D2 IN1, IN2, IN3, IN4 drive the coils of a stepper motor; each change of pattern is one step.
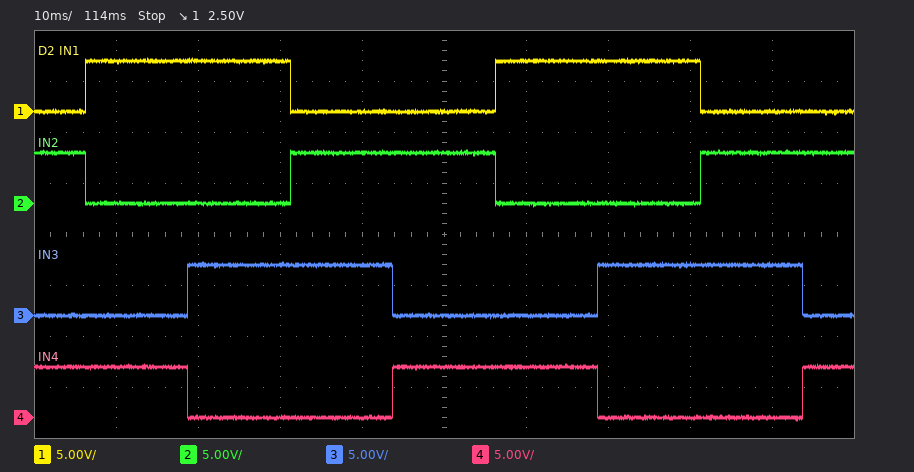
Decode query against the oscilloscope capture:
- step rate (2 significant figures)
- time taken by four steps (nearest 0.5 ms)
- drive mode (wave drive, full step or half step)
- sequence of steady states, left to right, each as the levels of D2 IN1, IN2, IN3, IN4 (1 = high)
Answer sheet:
80 steps/s
50.0 ms
full step
0101 1001 1010 0110 0101 1001 1010 0110 0101
